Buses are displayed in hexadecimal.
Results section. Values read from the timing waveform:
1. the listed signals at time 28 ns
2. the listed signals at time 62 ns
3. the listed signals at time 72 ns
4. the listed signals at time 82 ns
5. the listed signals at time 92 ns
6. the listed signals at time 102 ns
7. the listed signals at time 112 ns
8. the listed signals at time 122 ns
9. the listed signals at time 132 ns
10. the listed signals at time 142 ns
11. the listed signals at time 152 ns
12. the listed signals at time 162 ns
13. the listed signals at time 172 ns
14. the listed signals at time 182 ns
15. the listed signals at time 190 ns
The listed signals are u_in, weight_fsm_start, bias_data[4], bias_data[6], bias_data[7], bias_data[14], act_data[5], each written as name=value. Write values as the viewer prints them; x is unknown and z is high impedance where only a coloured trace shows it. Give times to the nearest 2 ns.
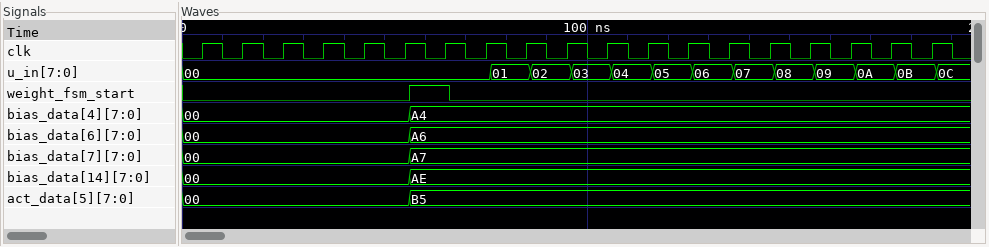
u_in=00, weight_fsm_start=0, bias_data[4]=00, bias_data[6]=00, bias_data[7]=00, bias_data[14]=00, act_data[5]=00
u_in=00, weight_fsm_start=1, bias_data[4]=A4, bias_data[6]=A6, bias_data[7]=A7, bias_data[14]=AE, act_data[5]=B5
u_in=00, weight_fsm_start=0, bias_data[4]=A4, bias_data[6]=A6, bias_data[7]=A7, bias_data[14]=AE, act_data[5]=B5
u_in=01, weight_fsm_start=0, bias_data[4]=A4, bias_data[6]=A6, bias_data[7]=A7, bias_data[14]=AE, act_data[5]=B5
u_in=02, weight_fsm_start=0, bias_data[4]=A4, bias_data[6]=A6, bias_data[7]=A7, bias_data[14]=AE, act_data[5]=B5
u_in=03, weight_fsm_start=0, bias_data[4]=A4, bias_data[6]=A6, bias_data[7]=A7, bias_data[14]=AE, act_data[5]=B5
u_in=04, weight_fsm_start=0, bias_data[4]=A4, bias_data[6]=A6, bias_data[7]=A7, bias_data[14]=AE, act_data[5]=B5
u_in=05, weight_fsm_start=0, bias_data[4]=A4, bias_data[6]=A6, bias_data[7]=A7, bias_data[14]=AE, act_data[5]=B5
u_in=06, weight_fsm_start=0, bias_data[4]=A4, bias_data[6]=A6, bias_data[7]=A7, bias_data[14]=AE, act_data[5]=B5
u_in=07, weight_fsm_start=0, bias_data[4]=A4, bias_data[6]=A6, bias_data[7]=A7, bias_data[14]=AE, act_data[5]=B5
u_in=08, weight_fsm_start=0, bias_data[4]=A4, bias_data[6]=A6, bias_data[7]=A7, bias_data[14]=AE, act_data[5]=B5
u_in=09, weight_fsm_start=0, bias_data[4]=A4, bias_data[6]=A6, bias_data[7]=A7, bias_data[14]=AE, act_data[5]=B5
u_in=0A, weight_fsm_start=0, bias_data[4]=A4, bias_data[6]=A6, bias_data[7]=A7, bias_data[14]=AE, act_data[5]=B5
u_in=0B, weight_fsm_start=0, bias_data[4]=A4, bias_data[6]=A6, bias_data[7]=A7, bias_data[14]=AE, act_data[5]=B5
u_in=0C, weight_fsm_start=0, bias_data[4]=A4, bias_data[6]=A6, bias_data[7]=A7, bias_data[14]=AE, act_data[5]=B5
